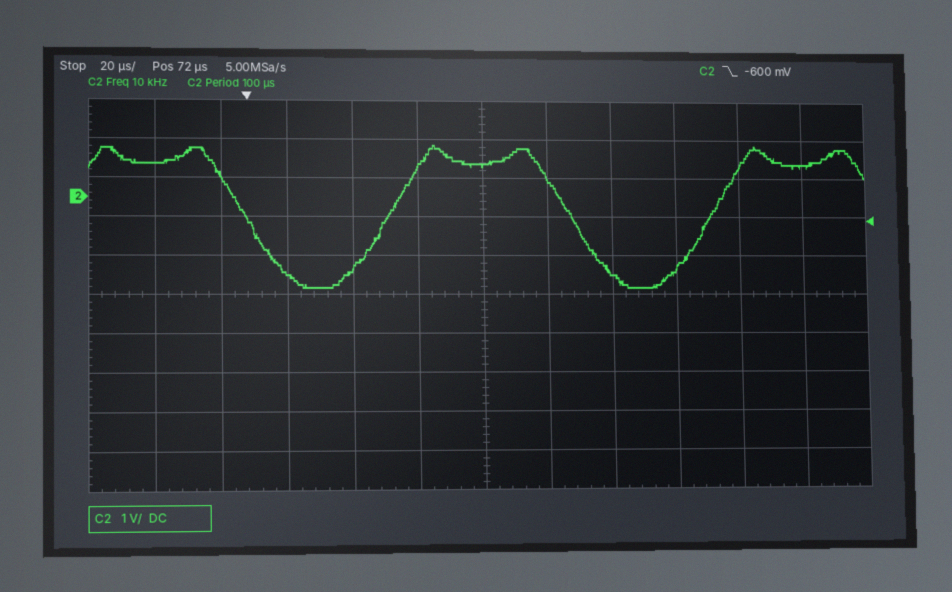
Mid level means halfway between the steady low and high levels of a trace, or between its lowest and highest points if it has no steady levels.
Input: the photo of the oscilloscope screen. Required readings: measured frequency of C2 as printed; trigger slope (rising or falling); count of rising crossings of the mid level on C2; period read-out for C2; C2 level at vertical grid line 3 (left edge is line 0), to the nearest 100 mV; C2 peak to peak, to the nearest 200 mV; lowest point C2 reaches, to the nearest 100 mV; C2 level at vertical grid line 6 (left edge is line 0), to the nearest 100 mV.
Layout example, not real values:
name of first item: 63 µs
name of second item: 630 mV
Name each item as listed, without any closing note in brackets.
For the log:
measured frequency of C2 as printed: 10 kHz
trigger slope: falling
count of rising crossings of the mid level on C2: 2
period read-out for C2: 100 µs
C2 level at vertical grid line 3 (left edge is line 0), to the nearest 100 mV: -2.0 V
C2 peak to peak, to the nearest 200 mV: 3.6 V
lowest point C2 reaches, to the nearest 100 mV: -2.3 V
C2 level at vertical grid line 6 (left edge is line 0), to the nearest 100 mV: 800 mV
